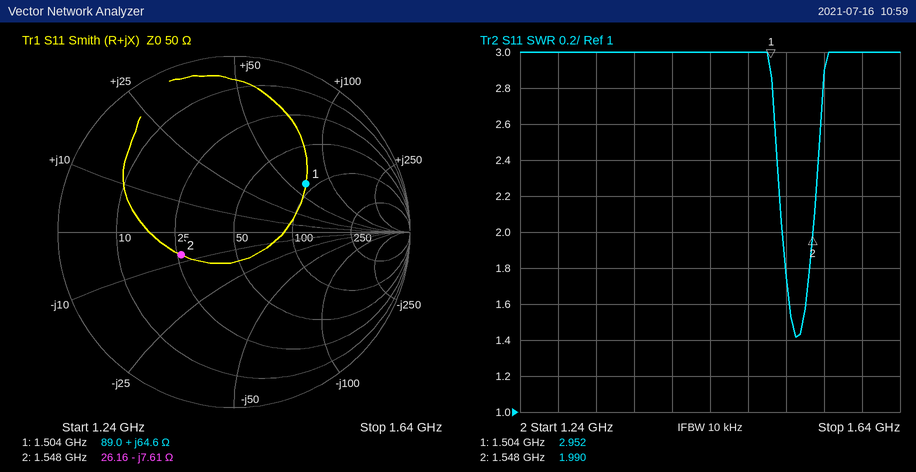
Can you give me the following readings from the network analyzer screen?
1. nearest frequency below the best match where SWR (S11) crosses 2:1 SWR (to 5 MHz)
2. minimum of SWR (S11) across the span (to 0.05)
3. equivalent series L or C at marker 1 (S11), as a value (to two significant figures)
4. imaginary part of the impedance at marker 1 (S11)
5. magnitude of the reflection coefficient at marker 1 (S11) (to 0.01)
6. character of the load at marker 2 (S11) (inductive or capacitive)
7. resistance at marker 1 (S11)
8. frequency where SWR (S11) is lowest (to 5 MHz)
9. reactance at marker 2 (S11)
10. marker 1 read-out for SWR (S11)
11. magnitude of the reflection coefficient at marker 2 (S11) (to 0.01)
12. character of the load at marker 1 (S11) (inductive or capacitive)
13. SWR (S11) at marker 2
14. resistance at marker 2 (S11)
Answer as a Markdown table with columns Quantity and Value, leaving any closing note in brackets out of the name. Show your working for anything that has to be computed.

| Quantity | Value |
|---|---|
| nearest frequency below the best match where SWR (S11) crosses 2:1 SWR | 1.515 GHz |
| minimum of SWR (S11) across the span | 1.40 |
| equivalent series L or C at marker 1 (S11), as a value | L = 64.6 Ω/(2π × 1.504 GHz) ≈ 6.8 nH |
| imaginary part of the impedance at marker 1 | +64.6 Ω |
| magnitude of the reflection coefficient at marker 1 (S11) | 0.49 |
| character of the load at marker 2 (S11) | capacitive |
| resistance at marker 1 | 89.0 Ω |
| frequency where SWR (S11) is lowest | 1.530 GHz |
| reactance at marker 2 | -7.61 Ω |
| marker 1 read-out for SWR | 2.952 |
| magnitude of the reflection coefficient at marker 2 (S11) | 0.33 |
| character of the load at marker 1 (S11) | inductive |
| SWR (S11) at marker 2 | 1.990 |
| resistance at marker 2 | 26.16 Ω |
